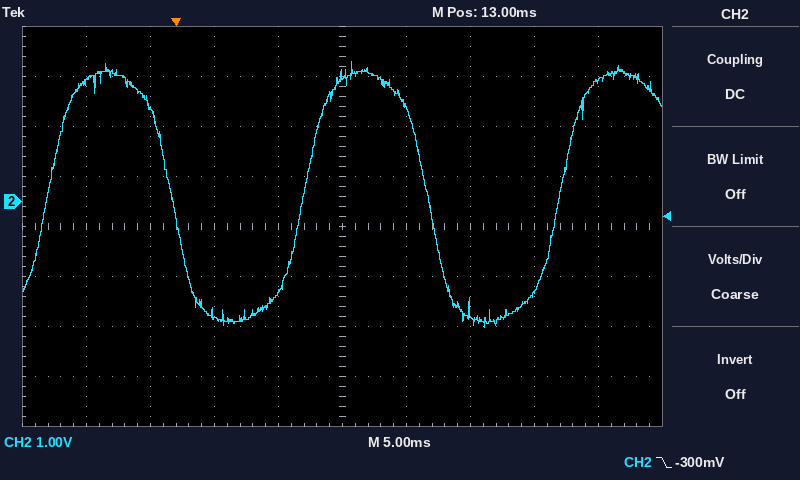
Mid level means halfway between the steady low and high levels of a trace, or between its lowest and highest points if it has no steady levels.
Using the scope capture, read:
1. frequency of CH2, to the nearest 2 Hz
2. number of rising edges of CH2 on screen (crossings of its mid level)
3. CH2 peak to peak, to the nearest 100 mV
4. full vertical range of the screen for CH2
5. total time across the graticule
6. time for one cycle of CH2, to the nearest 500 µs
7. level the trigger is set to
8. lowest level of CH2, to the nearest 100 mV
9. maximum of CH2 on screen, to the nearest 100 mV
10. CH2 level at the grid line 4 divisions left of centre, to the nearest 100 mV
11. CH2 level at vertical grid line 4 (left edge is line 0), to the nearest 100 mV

50 Hz
3
5.3 V
8 V
50 ms
20.0 ms
-300 mV
-2.5 V
2.8 V
2.4 V
-1.8 V
